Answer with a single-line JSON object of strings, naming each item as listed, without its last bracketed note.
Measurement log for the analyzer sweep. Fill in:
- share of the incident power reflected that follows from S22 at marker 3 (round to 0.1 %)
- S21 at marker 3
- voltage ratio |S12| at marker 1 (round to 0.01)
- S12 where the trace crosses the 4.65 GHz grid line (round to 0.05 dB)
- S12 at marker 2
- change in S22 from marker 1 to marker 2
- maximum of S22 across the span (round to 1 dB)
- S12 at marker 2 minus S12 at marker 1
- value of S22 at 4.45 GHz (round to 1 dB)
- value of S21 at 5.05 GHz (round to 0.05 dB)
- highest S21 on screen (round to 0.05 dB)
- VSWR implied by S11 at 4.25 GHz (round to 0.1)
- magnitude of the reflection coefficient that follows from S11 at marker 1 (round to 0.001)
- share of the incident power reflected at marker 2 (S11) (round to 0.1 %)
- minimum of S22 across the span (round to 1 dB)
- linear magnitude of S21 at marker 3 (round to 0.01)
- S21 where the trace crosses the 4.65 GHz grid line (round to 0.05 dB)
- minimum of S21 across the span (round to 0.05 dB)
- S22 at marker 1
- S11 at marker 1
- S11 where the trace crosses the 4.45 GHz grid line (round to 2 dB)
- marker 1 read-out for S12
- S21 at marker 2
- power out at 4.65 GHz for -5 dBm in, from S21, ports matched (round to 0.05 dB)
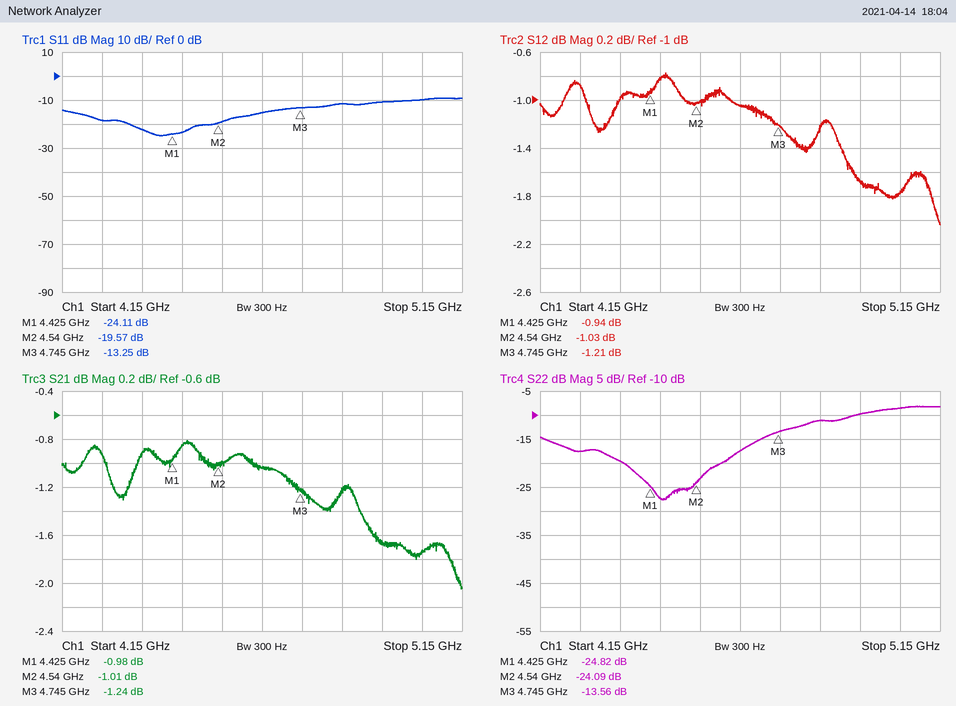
{"share of the incident power reflected that follows from S22 at marker 3": "4.4 %", "S21 at marker 3": "-1.24 dB", "voltage ratio |S12| at marker 1": "0.90", "S12 where the trace crosses the 4.65 GHz grid line": "-1.05 dB", "S12 at marker 2": "-1.03 dB", "change in S22 from marker 1 to marker 2": "0.73 dB", "maximum of S22 across the span": "-8 dB", "S12 at marker 2 minus S12 at marker 1": "-0.09 dB", "value of S22 at 4.45 GHz": "-27 dB", "value of S21 at 5.05 GHz": "-1.75 dB", "highest S21 on screen": "-0.80 dB", "VSWR implied by S11 at 4.25 GHz": "1.3", "magnitude of the reflection coefficient that follows from S11 at marker 1": "0.062", "share of the incident power reflected at marker 2 (S11)": "1.1 %", "minimum of S22 across the span": "-28 dB", "linear magnitude of S21 at marker 3": "0.87", "S21 where the trace crosses the 4.65 GHz grid line": "-1.05 dB", "minimum of S21 across the span": "-2.05 dB", "S22 at marker 1": "-24.82 dB", "S11 at marker 1": "-24.11 dB", "S11 where the trace crosses the 4.45 GHz grid line": "-24 dB", "marker 1 read-out for S12": "-0.94 dB", "S21 at marker 2": "-1.01 dB", "power out at 4.65 GHz for -5 dBm in, from S21, ports matched": "-6.05 dBm"}
